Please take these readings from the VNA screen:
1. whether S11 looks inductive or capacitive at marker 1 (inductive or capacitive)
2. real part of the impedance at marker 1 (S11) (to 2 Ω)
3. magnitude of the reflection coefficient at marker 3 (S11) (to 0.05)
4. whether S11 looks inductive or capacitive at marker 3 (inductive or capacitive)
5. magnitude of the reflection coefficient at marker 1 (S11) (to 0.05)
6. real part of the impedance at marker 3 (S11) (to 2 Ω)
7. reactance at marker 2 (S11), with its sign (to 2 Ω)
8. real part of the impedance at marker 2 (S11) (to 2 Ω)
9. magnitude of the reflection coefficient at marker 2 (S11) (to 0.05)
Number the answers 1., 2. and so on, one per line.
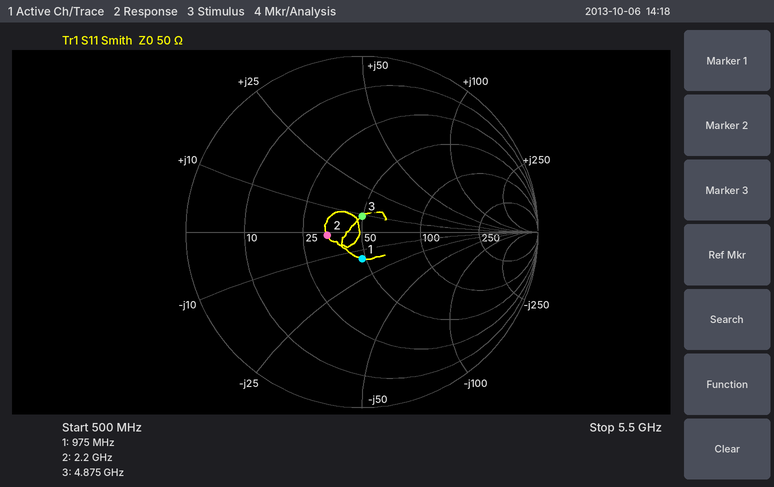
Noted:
1. capacitive
2. 48 Ω
3. 0.10
4. inductive
5. 0.15
6. 50 Ω
7. -2 Ω
8. 34 Ω
9. 0.20
